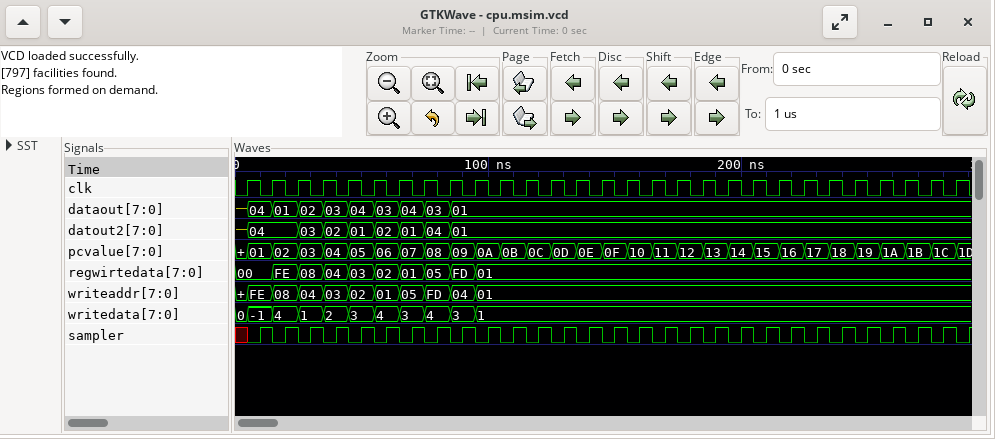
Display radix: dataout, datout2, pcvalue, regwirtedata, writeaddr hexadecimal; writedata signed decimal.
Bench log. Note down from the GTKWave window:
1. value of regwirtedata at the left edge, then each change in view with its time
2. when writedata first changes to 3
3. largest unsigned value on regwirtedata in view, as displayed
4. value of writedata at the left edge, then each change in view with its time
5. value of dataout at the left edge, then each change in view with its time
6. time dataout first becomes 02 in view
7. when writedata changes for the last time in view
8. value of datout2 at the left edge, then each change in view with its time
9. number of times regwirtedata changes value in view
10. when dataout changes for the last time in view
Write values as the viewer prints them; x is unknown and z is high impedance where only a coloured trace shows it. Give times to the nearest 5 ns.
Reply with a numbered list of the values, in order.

1. 00, FE at 15 ns, 08 at 25 ns, 04 at 35 ns, 03 at 45 ns, 02 at 55 ns, 01 at 65 ns, 05 at 75 ns, FD at 85 ns, 01 at 95 ns
2. 45 ns
3. FE
4. 0, -1 at 5 ns, 4 at 15 ns, 1 at 25 ns, 2 at 35 ns, 3 at 45 ns, 4 at 55 ns, 3 at 65 ns, 4 at 75 ns, 3 at 85 ns, 1 at 95 ns
5. z, 04 at 5 ns, 01 at 15 ns, 02 at 25 ns, 03 at 35 ns, 04 at 45 ns, 03 at 55 ns, 04 at 65 ns, 03 at 75 ns, 01 at 85 ns
6. 25 ns
7. 95 ns
8. z, 04 at 5 ns, 03 at 25 ns, 02 at 35 ns, 01 at 45 ns, 02 at 55 ns, 01 at 65 ns, 04 at 75 ns, 01 at 85 ns
9. 9
10. 85 ns
